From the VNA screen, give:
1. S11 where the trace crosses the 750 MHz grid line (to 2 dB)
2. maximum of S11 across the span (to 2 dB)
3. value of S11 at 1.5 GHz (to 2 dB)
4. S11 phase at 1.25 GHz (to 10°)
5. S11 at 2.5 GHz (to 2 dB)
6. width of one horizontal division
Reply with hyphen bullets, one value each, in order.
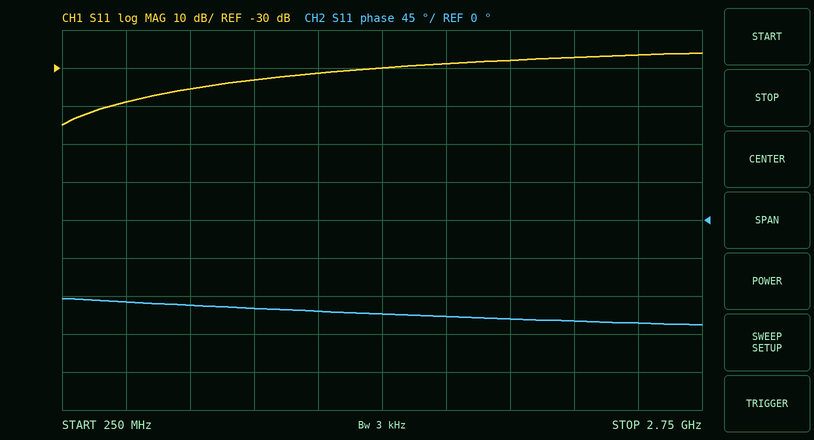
- -36 dB
- -26 dB
- -30 dB
- -110°
- -26 dB
- 250 MHz
